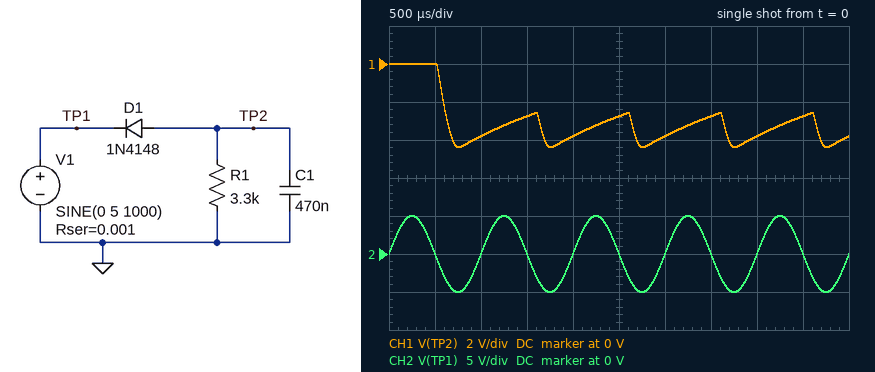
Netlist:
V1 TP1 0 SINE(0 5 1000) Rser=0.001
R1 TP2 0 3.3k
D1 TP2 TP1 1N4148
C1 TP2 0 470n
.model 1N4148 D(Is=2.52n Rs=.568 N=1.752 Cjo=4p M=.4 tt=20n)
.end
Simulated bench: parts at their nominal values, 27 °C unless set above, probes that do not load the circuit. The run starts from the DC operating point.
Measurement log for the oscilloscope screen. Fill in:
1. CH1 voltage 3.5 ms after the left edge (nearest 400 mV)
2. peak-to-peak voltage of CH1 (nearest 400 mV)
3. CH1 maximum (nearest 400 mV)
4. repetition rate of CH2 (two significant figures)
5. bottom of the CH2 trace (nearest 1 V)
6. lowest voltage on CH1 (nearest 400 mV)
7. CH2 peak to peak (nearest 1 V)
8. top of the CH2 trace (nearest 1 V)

-2.8 V
4.4 V
0 V
1.0 kHz
-5 V
-4.4 V
10 V
5 V
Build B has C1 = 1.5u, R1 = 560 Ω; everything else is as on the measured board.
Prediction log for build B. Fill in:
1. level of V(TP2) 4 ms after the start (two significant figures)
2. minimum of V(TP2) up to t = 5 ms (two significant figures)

-3.3 V
-4.3 V
